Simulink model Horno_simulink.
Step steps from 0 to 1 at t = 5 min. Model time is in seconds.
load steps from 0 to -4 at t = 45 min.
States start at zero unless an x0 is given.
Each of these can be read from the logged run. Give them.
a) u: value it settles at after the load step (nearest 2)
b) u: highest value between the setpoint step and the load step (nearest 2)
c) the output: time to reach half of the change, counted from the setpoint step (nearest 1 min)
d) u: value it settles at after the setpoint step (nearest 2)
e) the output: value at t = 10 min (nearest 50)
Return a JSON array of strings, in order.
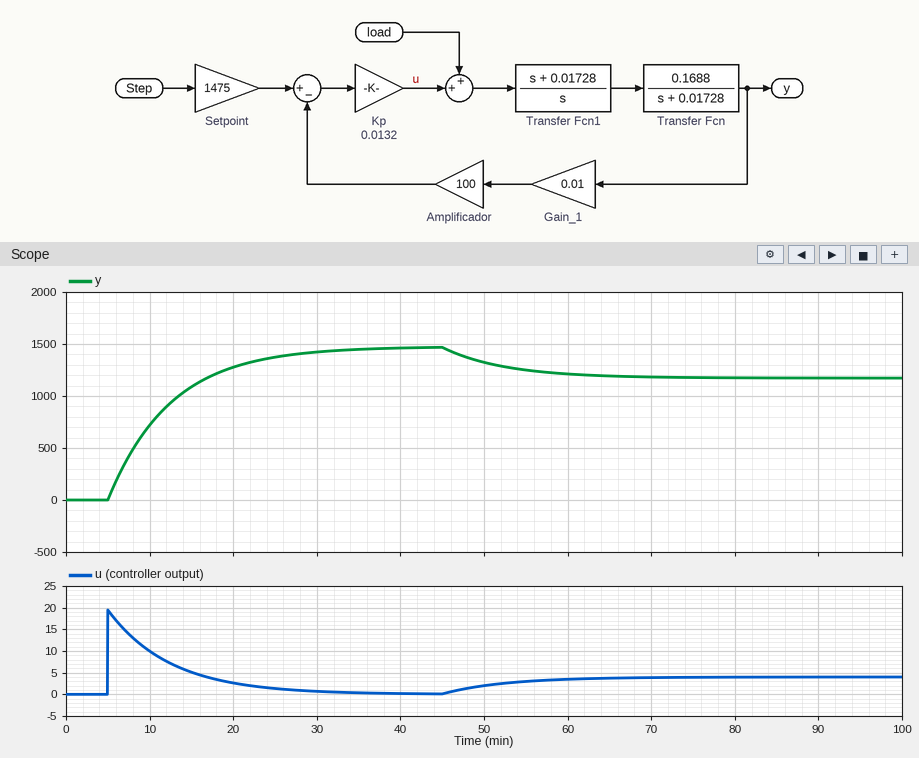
["4", "20", "5 min", "0", "700"]
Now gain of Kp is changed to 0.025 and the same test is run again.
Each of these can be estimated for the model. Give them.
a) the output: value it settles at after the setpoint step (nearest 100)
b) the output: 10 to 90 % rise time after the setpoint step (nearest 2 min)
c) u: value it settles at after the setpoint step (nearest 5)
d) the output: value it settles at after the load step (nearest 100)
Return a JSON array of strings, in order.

["1500", "8 min", "0", "1300"]
